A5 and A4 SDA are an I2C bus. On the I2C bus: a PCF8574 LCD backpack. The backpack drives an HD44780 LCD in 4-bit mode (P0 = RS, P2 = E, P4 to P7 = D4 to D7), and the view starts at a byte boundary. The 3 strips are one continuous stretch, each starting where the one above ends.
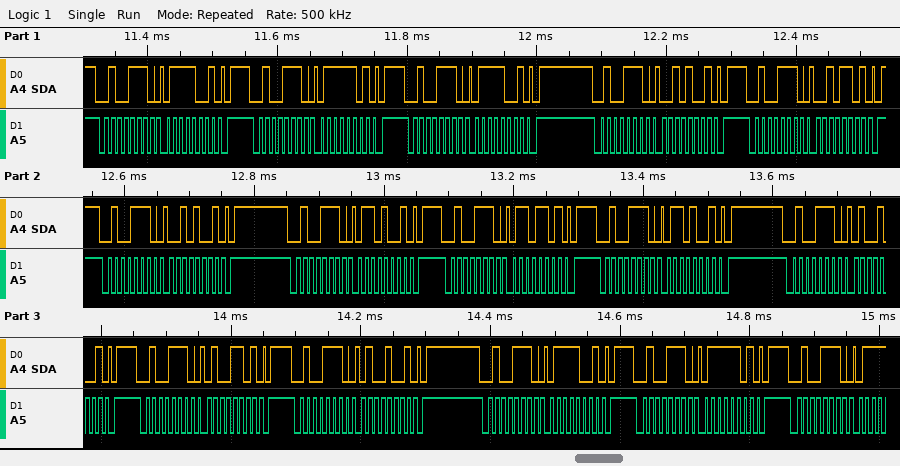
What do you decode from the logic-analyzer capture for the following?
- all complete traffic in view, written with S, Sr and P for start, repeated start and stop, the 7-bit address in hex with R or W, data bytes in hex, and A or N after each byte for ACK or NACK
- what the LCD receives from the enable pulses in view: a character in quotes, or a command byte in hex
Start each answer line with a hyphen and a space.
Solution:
- S 27W A 79 A P S 27W A 7D A P S 27W A 79 A P S 27W A 29 A P S 27W A 2D A P S 27W A 29 A P S 27W A 69 A P S 27W A 6D A P S 27W A 69 A P S 27W A 49 A P S 27W A 4D A P S 27W A 49 A P S 27W A 79 A P S 27W A 7D A P S 27W A
- 'r' 'd'
